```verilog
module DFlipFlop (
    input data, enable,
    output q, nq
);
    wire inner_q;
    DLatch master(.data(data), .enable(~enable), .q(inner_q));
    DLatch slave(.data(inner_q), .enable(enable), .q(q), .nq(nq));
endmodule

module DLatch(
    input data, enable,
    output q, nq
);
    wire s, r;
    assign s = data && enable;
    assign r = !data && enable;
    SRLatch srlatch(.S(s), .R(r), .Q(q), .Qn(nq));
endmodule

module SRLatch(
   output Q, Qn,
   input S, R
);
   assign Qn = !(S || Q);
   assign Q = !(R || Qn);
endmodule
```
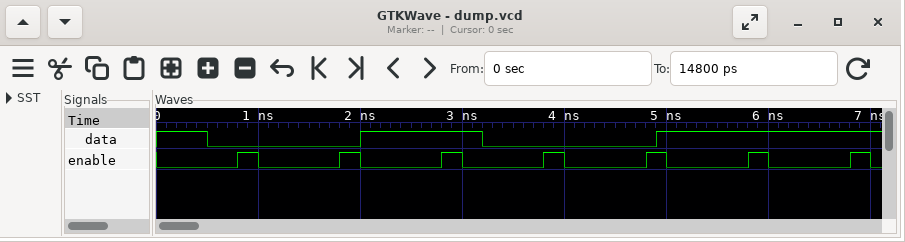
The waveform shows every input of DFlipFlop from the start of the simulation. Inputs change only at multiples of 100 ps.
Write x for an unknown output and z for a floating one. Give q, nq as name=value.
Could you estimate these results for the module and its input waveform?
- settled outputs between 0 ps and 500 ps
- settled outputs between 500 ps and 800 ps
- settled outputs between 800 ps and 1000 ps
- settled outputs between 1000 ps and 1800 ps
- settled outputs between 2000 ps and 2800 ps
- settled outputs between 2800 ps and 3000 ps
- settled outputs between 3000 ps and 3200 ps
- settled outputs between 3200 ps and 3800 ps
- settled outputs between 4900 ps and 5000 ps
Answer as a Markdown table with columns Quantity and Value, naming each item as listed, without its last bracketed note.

| Quantity | Value |
|---|---|
| settled outputs between 0 ps and 500 ps | q=x, nq=x |
| settled outputs between 500 ps and 800 ps | q=x, nq=x |
| settled outputs between 800 ps and 1000 ps | q=0, nq=1 |
| settled outputs between 1000 ps and 1800 ps | q=0, nq=1 |
| settled outputs between 2000 ps and 2800 ps | q=0, nq=1 |
| settled outputs between 2800 ps and 3000 ps | q=1, nq=0 |
| settled outputs between 3000 ps and 3200 ps | q=1, nq=0 |
| settled outputs between 3200 ps and 3800 ps | q=1, nq=0 |
| settled outputs between 4900 ps and 5000 ps | q=0, nq=1 |
